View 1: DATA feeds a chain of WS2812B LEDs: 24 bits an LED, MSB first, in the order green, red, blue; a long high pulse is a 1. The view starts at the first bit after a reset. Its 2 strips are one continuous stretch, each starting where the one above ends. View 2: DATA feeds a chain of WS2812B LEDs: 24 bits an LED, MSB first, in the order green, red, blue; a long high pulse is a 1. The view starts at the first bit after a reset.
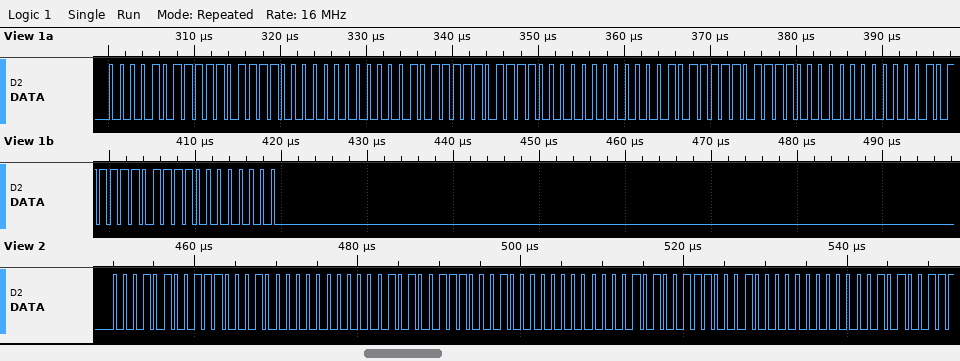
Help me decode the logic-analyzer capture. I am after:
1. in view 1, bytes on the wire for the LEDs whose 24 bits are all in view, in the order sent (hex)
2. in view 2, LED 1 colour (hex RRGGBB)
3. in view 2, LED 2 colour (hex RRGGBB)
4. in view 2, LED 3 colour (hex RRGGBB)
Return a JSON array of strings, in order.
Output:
["0B EF 00 0B EF 00 0B EF 00 0B EF 00", "#E21400", "#E21400", "#E21400"]
